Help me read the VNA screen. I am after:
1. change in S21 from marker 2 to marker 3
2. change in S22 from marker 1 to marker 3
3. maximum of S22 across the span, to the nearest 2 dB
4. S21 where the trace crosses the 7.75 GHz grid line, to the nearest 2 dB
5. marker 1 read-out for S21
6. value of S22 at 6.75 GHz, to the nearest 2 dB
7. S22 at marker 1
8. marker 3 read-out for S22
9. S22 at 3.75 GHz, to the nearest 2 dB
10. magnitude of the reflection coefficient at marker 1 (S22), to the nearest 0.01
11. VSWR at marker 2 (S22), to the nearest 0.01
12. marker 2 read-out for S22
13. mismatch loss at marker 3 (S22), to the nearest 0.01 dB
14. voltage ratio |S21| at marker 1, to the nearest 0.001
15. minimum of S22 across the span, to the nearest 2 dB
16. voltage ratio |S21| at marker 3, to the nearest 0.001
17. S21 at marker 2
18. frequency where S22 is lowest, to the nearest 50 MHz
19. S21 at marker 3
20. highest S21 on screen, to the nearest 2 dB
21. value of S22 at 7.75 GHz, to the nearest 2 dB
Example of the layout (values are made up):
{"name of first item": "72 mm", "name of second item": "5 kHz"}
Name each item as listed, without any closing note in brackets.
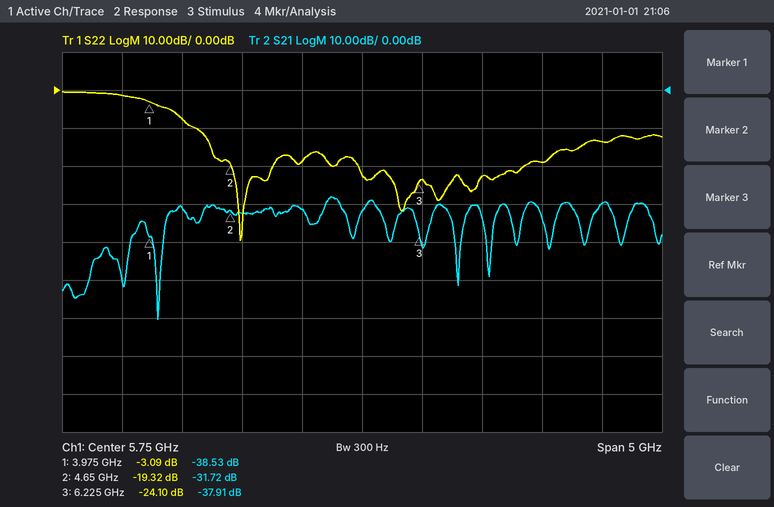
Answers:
{"change in S21 from marker 2 to marker 3": "-6.19 dB", "change in S22 from marker 1 to marker 3": "-21.01 dB", "maximum of S22 across the span, to the nearest 2 dB": "0 dB", "S21 where the trace crosses the 7.75 GHz grid line, to the nearest 2 dB": "-30 dB", "marker 1 read-out for S21": "-38.53 dB", "value of S22 at 6.75 GHz, to the nearest 2 dB": "-22 dB", "S22 at marker 1": "-3.09 dB", "marker 3 read-out for S22": "-24.10 dB", "S22 at 3.75 GHz, to the nearest 2 dB": "-2 dB", "magnitude of the reflection coefficient at marker 1 (S22), to the nearest 0.01": "0.70", "VSWR at marker 2 (S22), to the nearest 0.01": "1.24", "marker 2 read-out for S22": "-19.32 dB", "mismatch loss at marker 3 (S22), to the nearest 0.01 dB": "0.02 dB", "voltage ratio |S21| at marker 1, to the nearest 0.001": "0.012", "minimum of S22 across the span, to the nearest 2 dB": "-40 dB", "voltage ratio |S21| at marker 3, to the nearest 0.001": "0.013", "S21 at marker 2": "-31.72 dB", "frequency where S22 is lowest, to the nearest 50 MHz": "4.75 GHz", "S21 at marker 3": "-37.91 dB", "highest S21 on screen, to the nearest 2 dB": "-28 dB", "value of S22 at 7.75 GHz, to the nearest 2 dB": "-14 dB"}
